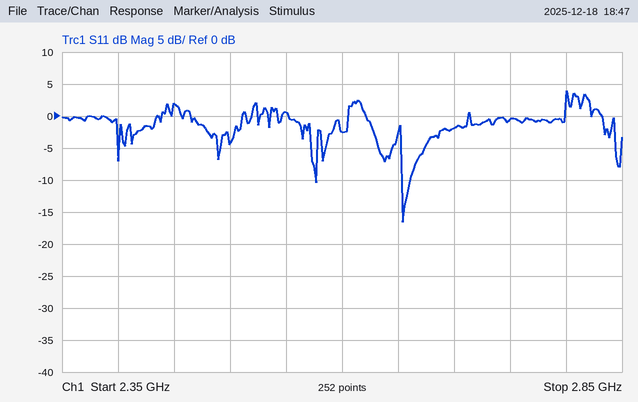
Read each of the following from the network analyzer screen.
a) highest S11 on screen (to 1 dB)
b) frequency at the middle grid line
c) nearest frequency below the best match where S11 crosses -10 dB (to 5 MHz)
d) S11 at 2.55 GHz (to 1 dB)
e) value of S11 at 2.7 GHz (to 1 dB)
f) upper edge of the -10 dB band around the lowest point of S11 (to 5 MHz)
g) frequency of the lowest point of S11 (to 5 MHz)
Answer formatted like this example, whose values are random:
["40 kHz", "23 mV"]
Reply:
["4 dB", "2.6 GHz", "2.655 GHz", "1 dB", "-2 dB", "2.660 GHz", "2.655 GHz"]
